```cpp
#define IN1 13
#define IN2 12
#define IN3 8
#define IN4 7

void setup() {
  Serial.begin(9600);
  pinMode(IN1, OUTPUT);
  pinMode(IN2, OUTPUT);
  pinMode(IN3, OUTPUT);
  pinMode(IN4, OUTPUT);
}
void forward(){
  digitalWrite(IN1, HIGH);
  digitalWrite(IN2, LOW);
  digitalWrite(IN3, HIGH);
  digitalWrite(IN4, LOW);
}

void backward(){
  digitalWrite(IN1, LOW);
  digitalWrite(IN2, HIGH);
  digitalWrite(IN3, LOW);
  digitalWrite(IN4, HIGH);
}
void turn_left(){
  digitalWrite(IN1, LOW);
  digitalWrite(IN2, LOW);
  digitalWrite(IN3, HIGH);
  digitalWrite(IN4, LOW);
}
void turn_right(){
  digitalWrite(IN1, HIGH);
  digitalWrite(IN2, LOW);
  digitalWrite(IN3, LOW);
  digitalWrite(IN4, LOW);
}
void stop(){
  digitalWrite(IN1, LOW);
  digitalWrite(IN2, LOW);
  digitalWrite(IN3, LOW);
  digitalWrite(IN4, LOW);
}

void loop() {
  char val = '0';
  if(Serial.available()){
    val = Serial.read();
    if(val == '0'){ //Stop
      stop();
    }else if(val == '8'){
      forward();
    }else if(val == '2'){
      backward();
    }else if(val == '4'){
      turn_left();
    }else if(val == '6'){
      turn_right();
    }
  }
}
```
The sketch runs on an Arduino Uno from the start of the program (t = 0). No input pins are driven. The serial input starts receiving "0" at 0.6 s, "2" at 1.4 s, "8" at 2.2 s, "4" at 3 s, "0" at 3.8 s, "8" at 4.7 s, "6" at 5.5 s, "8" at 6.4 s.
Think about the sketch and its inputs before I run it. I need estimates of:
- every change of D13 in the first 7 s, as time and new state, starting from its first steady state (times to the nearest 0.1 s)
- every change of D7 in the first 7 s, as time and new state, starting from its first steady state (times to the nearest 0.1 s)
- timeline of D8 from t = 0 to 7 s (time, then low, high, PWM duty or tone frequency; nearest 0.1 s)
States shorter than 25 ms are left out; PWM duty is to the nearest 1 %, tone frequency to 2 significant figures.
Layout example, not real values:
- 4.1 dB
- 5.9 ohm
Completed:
- 0 s low; 2.2 s high; 3 s low; 4.7 s high
- 0 s low; 1.4 s high; 2.2 s low
- 0 s low; 2.2 s high; 3.8 s low; 4.7 s high; 5.5 s low; 6.4 s high
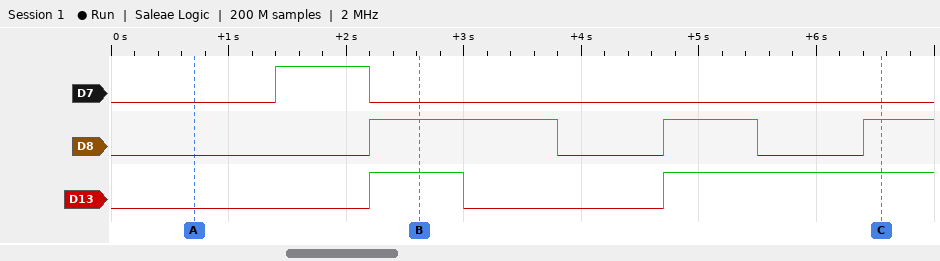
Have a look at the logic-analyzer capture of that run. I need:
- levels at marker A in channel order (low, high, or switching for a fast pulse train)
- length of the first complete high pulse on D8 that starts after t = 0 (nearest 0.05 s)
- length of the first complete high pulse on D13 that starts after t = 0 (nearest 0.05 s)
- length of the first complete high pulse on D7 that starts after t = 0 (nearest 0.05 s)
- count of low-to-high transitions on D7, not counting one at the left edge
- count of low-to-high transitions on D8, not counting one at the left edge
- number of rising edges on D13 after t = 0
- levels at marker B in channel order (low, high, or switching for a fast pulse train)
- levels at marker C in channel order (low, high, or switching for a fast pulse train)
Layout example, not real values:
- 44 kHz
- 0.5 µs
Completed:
- D7 low, D8 low, D13 low
- 1.60 s
- 0.80 s
- 0.80 s
- 1
- 3
- 2
- D7 low, D8 high, D13 high
- D7 low, D8 high, D13 high
